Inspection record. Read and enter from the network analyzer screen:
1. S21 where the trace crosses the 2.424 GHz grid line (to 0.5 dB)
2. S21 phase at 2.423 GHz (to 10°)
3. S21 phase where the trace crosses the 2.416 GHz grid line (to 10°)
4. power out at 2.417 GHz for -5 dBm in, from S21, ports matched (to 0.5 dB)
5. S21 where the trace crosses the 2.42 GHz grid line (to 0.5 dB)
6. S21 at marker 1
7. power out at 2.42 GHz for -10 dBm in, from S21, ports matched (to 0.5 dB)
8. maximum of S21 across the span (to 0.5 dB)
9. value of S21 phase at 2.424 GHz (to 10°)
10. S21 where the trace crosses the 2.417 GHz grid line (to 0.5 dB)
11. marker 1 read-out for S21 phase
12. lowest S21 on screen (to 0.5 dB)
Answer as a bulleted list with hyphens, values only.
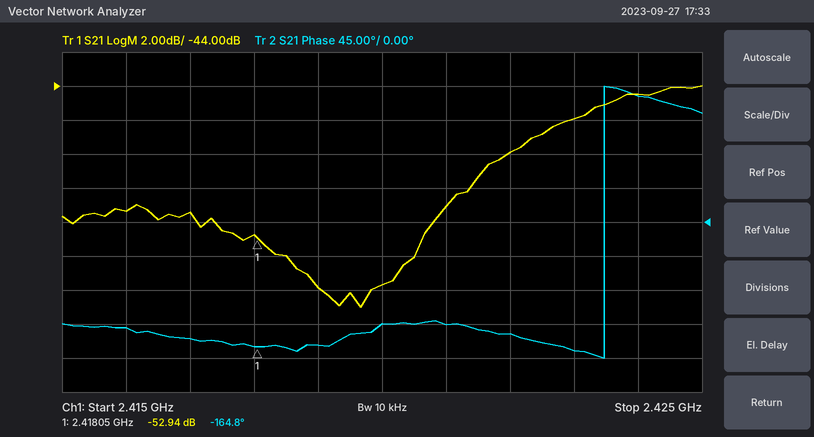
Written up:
- -44.5 dB
- -170°
- -140°
- -56.5 dBm
- -55.5 dB
- -52.94 dB
- -65.5 dBm
- -44.0 dB
- 170°
- -51.5 dB
- -164.8°
- -57.0 dB
